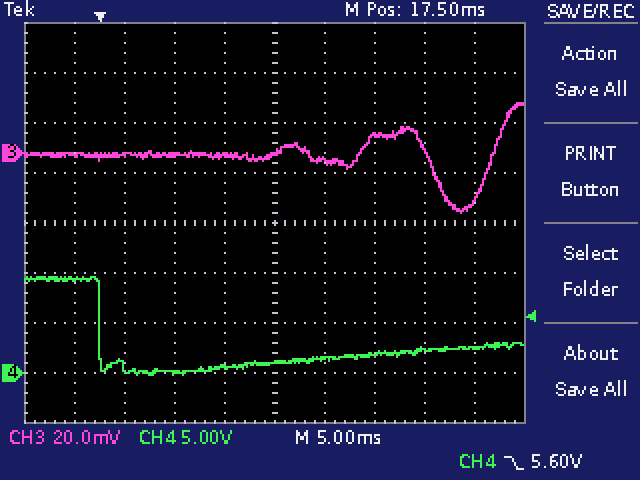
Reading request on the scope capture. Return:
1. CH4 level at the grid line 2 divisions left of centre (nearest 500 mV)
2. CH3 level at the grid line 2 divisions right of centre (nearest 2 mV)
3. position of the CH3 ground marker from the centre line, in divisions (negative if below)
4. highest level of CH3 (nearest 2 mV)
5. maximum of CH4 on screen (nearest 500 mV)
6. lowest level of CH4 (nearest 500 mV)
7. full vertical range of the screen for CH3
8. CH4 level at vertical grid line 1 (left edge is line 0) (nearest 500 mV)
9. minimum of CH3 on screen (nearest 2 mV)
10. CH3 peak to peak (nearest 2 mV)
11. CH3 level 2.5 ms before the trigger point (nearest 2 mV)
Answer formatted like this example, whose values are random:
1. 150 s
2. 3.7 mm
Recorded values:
1. 0.0 V
2. 8 mV
3. +1.4 div
4. 20 mV
5. 9.5 V
6. 0.0 V
7. 160 mV
8. 9.5 V
9. -24 mV
10. 44 mV
11. 0 mV
